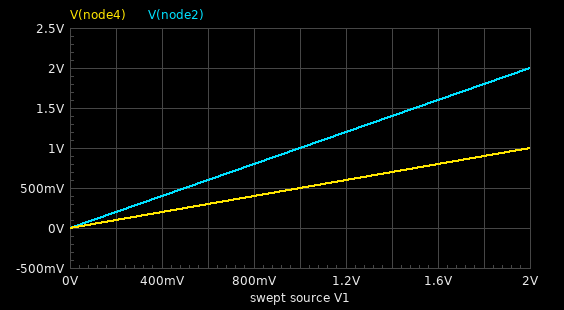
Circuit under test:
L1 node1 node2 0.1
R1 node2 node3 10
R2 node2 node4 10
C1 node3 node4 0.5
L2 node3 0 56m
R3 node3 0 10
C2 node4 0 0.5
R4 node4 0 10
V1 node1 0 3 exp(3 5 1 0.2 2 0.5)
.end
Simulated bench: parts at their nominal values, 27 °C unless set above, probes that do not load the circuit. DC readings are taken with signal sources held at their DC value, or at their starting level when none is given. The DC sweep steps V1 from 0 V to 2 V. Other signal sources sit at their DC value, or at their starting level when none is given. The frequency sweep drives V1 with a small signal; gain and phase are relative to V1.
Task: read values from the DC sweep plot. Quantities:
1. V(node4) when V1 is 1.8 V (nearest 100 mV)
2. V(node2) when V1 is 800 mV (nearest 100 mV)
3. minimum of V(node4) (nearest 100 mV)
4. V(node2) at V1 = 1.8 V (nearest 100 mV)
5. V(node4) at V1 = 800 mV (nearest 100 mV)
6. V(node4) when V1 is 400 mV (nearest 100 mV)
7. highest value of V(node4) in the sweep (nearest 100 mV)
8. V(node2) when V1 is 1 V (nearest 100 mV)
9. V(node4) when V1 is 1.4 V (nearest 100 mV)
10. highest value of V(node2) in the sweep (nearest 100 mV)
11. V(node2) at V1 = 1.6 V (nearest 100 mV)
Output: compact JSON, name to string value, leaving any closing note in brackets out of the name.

{"V(node4) when V1 is 1.8 V": "900 mV", "V(node2) when V1 is 800 mV": "800 mV", "minimum of V(node4)": "0 V", "V(node2) at V1 = 1.8 V": "1.8 V", "V(node4) at V1 = 800 mV": "400 mV", "V(node4) when V1 is 400 mV": "200 mV", "highest value of V(node4) in the sweep": "1.0 V", "V(node2) when V1 is 1 V": "1.0 V", "V(node4) when V1 is 1.4 V": "700 mV", "highest value of V(node2) in the sweep": "2.0 V", "V(node2) at V1 = 1.6 V": "1.6 V"}
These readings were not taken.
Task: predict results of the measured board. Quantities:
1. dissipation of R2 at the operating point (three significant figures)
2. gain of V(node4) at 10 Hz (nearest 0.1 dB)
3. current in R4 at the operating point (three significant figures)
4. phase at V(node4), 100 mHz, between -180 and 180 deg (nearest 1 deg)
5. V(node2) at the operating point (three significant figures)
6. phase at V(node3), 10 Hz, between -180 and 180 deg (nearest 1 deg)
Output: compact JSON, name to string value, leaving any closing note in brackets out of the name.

{"dissipation of R2 at the operating point": "225 mW", "gain of V(node4) at 10 Hz": "-47.9 dB", "current in R4 at the operating point": "150 mA", "phase at V(node4), 100 mHz, between -180 and 180 deg": "-73 deg", "V(node2) at the operating point": "3.00 V", "phase at V(node3), 10 Hz, between -180 and 180 deg": "-141 deg"}
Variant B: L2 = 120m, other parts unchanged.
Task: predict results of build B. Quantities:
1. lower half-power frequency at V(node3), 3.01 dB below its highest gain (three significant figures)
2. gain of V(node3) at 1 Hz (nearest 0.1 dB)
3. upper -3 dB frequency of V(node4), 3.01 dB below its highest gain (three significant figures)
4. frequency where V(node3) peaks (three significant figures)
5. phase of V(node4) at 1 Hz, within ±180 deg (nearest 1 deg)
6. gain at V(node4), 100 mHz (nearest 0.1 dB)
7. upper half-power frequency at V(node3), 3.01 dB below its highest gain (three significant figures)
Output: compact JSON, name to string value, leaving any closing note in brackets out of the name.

{"lower half-power frequency at V(node3), 3.01 dB below its highest gain": "846 mHz", "gain of V(node3) at 1 Hz": "-7.2 dB", "upper -3 dB frequency of V(node4), 3.01 dB below its highest gain": "31.7 mHz", "frequency where V(node3) peaks": "922 mHz", "phase of V(node4) at 1 Hz, within ±180 deg": "-51 deg", "gain at V(node4), 100 mHz": "-16.7 dB", "upper half-power frequency at V(node3), 3.01 dB below its highest gain": "1.01 Hz"}
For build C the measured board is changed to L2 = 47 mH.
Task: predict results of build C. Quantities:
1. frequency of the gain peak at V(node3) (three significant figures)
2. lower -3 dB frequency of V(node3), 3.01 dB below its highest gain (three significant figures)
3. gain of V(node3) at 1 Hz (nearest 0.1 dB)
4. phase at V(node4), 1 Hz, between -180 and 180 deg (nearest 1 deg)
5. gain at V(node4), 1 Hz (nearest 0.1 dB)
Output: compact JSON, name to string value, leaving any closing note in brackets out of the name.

{"frequency of the gain peak at V(node3)": "1.47 Hz", "lower -3 dB frequency of V(node3), 3.01 dB below its highest gain": "1.40 Hz", "gain of V(node3) at 1 Hz": "-21.9 dB", "phase at V(node4), 1 Hz, between -180 and 180 deg": "73 deg", "gain at V(node4), 1 Hz": "-32.1 dB"}
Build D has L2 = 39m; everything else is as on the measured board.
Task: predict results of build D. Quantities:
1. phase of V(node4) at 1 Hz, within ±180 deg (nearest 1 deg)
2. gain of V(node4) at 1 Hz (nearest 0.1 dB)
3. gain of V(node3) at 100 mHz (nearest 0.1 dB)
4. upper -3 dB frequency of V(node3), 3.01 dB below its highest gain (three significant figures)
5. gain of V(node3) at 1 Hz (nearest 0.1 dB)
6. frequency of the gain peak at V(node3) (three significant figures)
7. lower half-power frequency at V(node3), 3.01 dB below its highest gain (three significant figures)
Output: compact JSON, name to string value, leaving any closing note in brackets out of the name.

{"phase of V(node4) at 1 Hz, within ±180 deg": "74 deg", "gain of V(node4) at 1 Hz": "-37.2 dB", "gain of V(node3) at 100 mHz": "-48.9 dB", "upper -3 dB frequency of V(node3), 3.01 dB below its highest gain": "1.70 Hz", "gain of V(node3) at 1 Hz": "-24.6 dB", "frequency of the gain peak at V(node3)": "1.62 Hz", "lower half-power frequency at V(node3), 3.01 dB below its highest gain": "1.54 Hz"}
